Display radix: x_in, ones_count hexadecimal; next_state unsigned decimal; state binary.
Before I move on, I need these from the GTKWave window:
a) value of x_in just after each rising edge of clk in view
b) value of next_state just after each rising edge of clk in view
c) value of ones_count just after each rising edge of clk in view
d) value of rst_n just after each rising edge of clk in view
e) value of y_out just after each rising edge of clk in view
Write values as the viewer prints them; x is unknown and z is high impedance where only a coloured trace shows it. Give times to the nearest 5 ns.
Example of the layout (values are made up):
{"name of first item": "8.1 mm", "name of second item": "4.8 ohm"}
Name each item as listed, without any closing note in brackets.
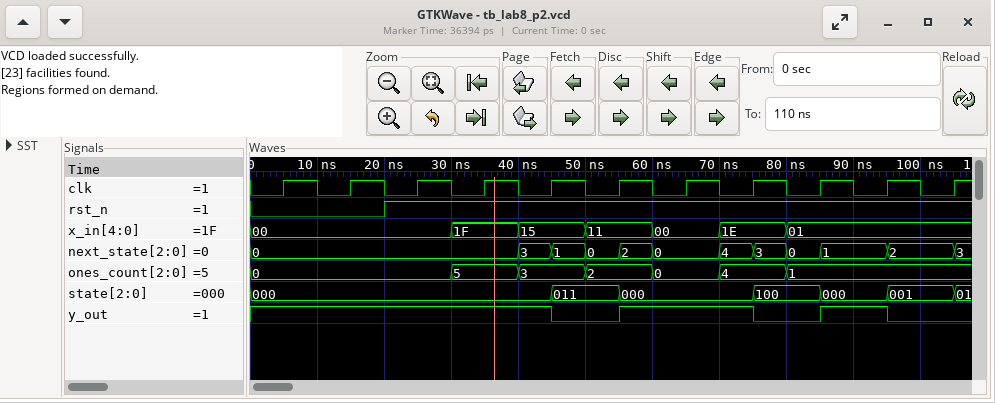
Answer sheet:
{"value of x_in just after each rising edge of clk in view": "00, 00, 00, 1F, 15, 11, 00, 1E, 01, 01, 01", "value of next_state just after each rising edge of clk in view": "0, 0, 0, 0, 1, 2, 0, 3, 1, 2, 3", "value of ones_count just after each rising edge of clk in view": "0, 0, 0, 5, 3, 2, 0, 4, 1, 1, 1", "value of rst_n just after each rising edge of clk in view": "0 0 1 1 1 1 1 1 1 1 1", "value of y_out just after each rising edge of clk in view": "1 1 1 1 0 1 1 0 1 0 0"}
